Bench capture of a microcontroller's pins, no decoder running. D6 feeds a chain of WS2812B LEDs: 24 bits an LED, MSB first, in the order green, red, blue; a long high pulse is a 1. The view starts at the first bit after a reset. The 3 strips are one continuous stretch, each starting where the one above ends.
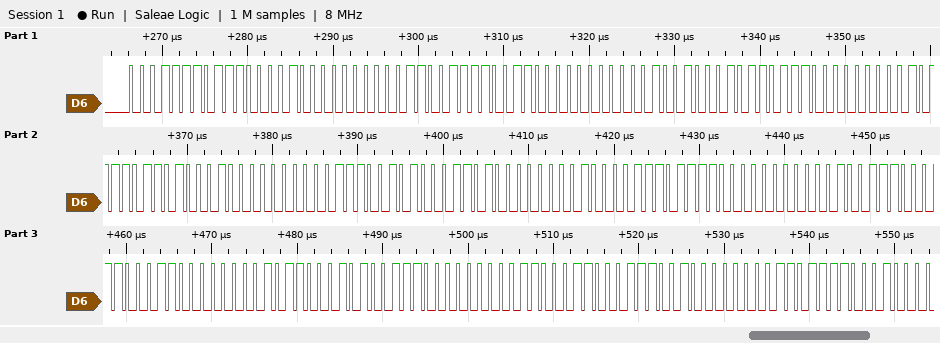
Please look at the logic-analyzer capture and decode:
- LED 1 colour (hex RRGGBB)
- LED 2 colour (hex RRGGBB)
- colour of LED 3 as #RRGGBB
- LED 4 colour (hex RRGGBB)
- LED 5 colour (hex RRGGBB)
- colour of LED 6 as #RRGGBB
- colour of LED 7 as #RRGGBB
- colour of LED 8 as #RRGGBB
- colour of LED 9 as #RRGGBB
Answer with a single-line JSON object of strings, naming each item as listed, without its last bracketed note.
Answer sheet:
{"LED 1 colour": "#E11E00", "LED 2 colour": "#CC3300", "colour of LED 3 as #RRGGBB": "#B74800", "LED 4 colour": "#A25D00", "LED 5 colour": "#8D7200", "colour of LED 6 as #RRGGBB": "#788700", "colour of LED 7 as #RRGGBB": "#639C00", "colour of LED 8 as #RRGGBB": "#4EB100", "colour of LED 9 as #RRGGBB": "#39C600"}
